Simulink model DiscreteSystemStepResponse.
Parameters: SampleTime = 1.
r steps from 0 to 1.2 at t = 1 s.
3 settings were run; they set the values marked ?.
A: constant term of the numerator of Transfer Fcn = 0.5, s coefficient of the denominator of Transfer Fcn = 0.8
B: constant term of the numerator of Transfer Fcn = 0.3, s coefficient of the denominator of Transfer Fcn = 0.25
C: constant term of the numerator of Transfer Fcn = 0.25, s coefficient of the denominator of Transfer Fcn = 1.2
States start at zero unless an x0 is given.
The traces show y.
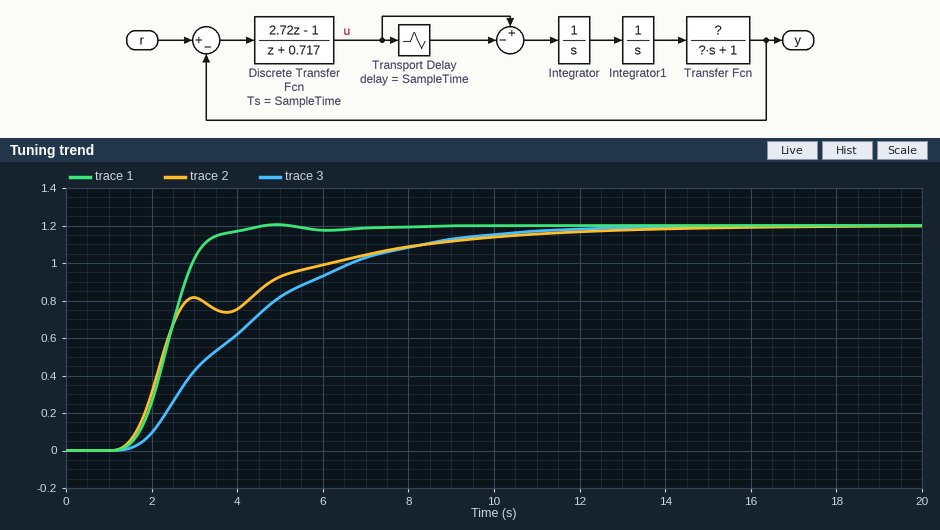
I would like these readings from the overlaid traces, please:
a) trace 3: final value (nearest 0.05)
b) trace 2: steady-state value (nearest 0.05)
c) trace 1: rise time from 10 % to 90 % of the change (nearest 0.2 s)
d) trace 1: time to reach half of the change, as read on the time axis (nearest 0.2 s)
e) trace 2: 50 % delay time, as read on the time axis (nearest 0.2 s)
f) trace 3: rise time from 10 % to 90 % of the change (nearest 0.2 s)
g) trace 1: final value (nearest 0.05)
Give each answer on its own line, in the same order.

1.20
1.20
1.4 s
2.4 s
2.4 s
5.8 s
1.20
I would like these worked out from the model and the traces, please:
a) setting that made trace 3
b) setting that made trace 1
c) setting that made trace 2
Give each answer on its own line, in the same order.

C
A
B
